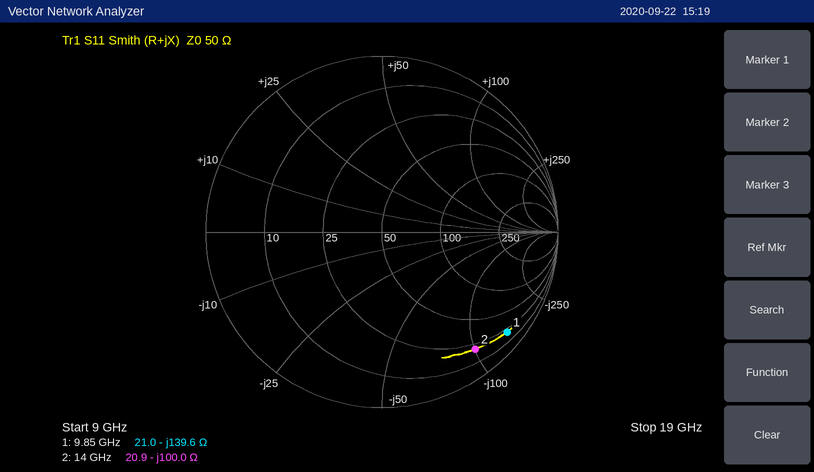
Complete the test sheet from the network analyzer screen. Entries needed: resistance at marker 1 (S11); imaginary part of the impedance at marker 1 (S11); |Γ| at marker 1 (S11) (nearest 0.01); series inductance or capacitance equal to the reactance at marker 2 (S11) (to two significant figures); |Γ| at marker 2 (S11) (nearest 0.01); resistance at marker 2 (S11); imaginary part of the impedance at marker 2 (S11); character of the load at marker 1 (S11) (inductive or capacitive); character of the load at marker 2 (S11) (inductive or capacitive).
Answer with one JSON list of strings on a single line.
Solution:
["21.0 Ω", "-139.6 Ω", "0.91", "110 fF", "0.85", "20.9 Ω", "-100.0 Ω", "capacitive", "capacitive"]
